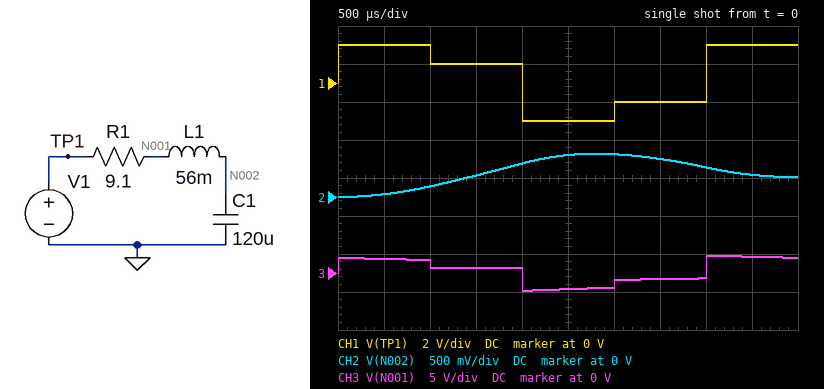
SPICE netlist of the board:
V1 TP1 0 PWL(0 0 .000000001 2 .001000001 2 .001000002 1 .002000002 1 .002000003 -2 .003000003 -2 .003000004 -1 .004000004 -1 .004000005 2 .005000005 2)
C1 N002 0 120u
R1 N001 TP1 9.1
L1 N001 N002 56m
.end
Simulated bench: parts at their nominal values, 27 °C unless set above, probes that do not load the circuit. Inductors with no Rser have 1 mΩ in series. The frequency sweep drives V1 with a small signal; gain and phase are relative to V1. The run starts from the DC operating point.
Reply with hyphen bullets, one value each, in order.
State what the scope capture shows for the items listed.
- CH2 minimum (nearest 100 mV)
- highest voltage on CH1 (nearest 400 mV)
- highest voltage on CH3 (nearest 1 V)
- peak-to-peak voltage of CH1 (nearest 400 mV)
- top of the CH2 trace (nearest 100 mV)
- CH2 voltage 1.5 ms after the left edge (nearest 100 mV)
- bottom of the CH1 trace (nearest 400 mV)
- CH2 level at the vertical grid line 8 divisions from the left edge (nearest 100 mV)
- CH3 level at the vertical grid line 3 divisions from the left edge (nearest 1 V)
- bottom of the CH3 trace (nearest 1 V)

- 0 V
- 2.0 V
- 2 V
- 4.0 V
- 600 mV
- 300 mV
- -2.0 V
- 400 mV
- 1 V
- -2 V
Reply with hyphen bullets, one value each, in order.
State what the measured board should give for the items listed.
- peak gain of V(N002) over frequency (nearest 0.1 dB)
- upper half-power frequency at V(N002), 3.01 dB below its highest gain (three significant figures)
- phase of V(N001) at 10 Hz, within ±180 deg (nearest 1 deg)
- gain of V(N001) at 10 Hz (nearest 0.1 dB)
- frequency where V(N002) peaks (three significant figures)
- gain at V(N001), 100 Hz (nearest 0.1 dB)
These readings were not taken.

- 7.7 dB
- 70.6 Hz
- -4 deg
- 0 dB
- 58.6 Hz
- -0.7 dB
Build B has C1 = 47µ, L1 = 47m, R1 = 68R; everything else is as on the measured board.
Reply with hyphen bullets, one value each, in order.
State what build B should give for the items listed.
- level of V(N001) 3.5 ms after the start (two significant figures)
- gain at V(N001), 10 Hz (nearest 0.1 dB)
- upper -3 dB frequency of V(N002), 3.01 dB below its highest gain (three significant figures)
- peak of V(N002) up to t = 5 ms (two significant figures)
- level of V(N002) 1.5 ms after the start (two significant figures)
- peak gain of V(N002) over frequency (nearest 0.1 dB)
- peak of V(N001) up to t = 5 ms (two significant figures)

- 460 mV
- -0.2 dB
- 62.2 Hz
- 620 mV
- 470 mV
- 0 dB
- 3.2 V
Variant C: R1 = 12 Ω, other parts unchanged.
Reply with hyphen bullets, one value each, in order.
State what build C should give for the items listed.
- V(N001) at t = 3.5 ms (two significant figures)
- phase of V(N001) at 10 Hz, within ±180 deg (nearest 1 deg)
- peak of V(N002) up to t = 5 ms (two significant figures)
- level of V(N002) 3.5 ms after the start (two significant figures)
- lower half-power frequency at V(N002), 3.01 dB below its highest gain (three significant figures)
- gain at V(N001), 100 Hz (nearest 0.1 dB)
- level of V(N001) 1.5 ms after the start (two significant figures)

- -730 mV
- -5 deg
- 540 mV
- 460 mV
- 34.3 Hz
- -1.1 dB
- 580 mV
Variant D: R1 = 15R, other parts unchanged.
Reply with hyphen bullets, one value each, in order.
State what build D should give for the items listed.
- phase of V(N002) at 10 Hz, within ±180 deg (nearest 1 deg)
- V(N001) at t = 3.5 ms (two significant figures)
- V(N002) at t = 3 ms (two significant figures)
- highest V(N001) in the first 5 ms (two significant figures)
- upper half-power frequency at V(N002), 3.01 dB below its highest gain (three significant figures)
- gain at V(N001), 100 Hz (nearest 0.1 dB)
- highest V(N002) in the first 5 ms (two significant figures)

- -7 deg
- -650 mV
- 500 mV
- 2.5 V
- 72.9 Hz
- -1.7 dB
- 510 mV
